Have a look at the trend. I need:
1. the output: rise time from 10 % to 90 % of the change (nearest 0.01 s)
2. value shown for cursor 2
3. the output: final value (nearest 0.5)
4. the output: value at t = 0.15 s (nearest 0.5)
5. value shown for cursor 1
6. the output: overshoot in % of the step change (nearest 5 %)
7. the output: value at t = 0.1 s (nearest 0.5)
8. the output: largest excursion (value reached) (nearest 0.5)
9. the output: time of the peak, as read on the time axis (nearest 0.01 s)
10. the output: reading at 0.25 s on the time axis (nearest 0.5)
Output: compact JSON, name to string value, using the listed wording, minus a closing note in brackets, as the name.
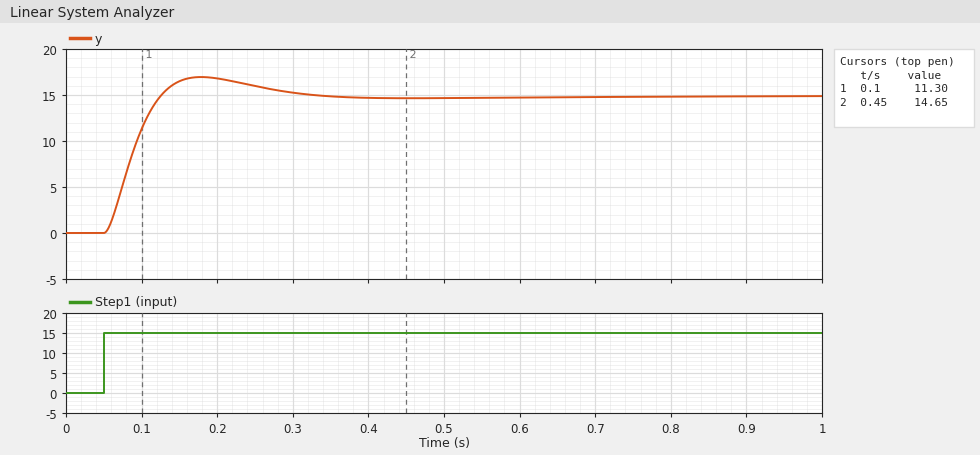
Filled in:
{"the output: rise time from 10 % to 90 % of the change": "0.05 s", "value shown for cursor 2": "14.65", "the output: final value": "15.0", "the output: value at t = 0.15 s": "16.5", "value shown for cursor 1": "11.30", "the output: overshoot in % of the step change": "15 %", "the output: value at t = 0.1 s": "11.5", "the output: largest excursion (value reached)": "17.0", "the output: time of the peak, as read on the time axis": "0.18 s", "the output: reading at 0.25 s on the time axis": "16.0"}
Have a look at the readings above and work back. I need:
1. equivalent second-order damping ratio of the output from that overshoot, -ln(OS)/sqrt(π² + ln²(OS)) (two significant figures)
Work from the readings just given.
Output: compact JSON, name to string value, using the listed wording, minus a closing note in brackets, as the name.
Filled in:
{"equivalent second-order damping ratio of the output from that overshoot, -ln(OS)/sqrt(π² + ln²(OS))": "0.52"}
